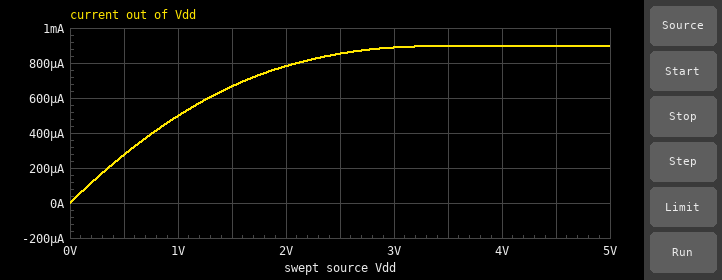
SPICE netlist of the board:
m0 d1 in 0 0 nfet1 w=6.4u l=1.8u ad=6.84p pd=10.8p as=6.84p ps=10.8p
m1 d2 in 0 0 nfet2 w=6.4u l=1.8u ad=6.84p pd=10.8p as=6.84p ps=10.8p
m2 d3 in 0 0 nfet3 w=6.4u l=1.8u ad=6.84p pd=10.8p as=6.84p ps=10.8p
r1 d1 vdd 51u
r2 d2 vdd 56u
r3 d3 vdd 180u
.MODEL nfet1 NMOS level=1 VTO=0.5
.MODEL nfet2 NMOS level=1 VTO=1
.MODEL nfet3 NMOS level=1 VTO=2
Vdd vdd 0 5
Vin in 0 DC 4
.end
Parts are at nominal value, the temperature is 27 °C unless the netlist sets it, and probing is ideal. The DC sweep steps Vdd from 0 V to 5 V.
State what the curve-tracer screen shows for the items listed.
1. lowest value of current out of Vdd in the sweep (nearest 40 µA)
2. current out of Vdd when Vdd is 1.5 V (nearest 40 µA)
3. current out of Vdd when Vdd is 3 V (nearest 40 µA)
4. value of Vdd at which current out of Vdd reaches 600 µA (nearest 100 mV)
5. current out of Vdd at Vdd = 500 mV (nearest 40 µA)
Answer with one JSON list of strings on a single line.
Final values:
["0 A", "680 µA", "880 µA", "1.3 V", "280 µA"]
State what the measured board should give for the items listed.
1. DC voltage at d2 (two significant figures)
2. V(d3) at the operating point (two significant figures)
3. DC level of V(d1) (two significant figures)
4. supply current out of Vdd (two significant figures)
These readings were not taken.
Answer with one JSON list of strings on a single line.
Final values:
["5.0 V", "5.0 V", "5.0 V", "900 µA"]
